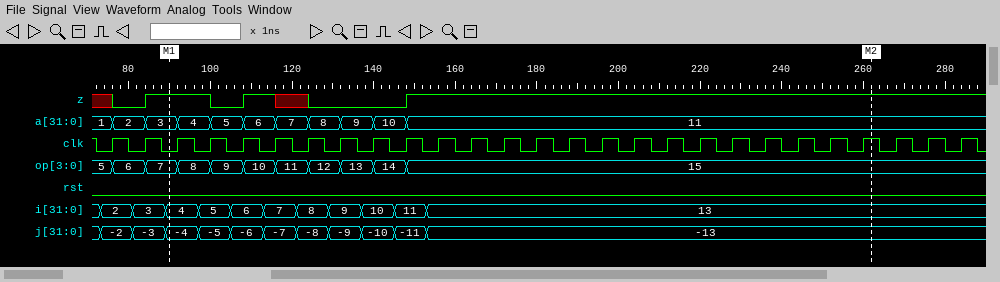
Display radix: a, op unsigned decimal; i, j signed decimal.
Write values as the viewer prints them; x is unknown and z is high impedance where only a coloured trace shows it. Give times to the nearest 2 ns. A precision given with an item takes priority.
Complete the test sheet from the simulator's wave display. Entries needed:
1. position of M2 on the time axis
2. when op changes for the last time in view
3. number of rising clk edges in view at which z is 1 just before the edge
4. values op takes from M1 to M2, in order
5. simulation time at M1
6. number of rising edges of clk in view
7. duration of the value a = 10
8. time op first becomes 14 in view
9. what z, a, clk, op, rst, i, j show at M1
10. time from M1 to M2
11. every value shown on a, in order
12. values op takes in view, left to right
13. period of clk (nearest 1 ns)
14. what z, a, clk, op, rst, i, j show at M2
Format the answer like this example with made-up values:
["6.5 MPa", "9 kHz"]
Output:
["262 ns", "148 ns", "20", "7, 8, 9, 10, 11, 12, 13, 14, 15", "90 ns", "27", "8 ns", "140 ns", "z=1, a=3, clk=0, op=7, rst=0, i=4, j=-4", "172 ns", "1, 2, 3, 4, 5, 6, 7, 8, 9, 10, 11", "5, 6, 7, 8, 9, 10, 11, 12, 13, 14, 15", "8 ns", "z=1, a=11, clk=1, op=15, rst=0, i=13, j=-13"]
